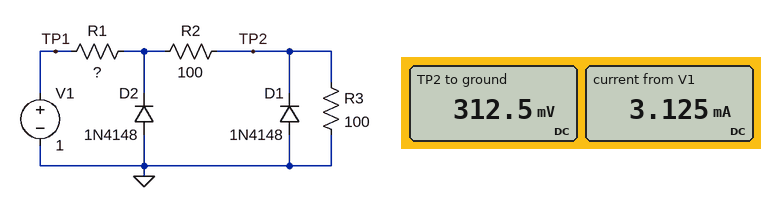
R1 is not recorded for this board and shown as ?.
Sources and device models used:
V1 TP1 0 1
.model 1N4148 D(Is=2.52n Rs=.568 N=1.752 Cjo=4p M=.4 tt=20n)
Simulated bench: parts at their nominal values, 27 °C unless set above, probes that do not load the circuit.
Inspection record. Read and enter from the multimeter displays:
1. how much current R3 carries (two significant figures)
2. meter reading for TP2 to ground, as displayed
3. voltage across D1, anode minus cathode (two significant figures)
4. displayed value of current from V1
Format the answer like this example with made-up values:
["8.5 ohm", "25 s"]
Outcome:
["3.1 mA", "312.5 mV", "-310 mV", "3.125 mA"]
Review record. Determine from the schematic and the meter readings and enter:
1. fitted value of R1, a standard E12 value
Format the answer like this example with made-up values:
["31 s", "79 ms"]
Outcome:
["120 Ω"]
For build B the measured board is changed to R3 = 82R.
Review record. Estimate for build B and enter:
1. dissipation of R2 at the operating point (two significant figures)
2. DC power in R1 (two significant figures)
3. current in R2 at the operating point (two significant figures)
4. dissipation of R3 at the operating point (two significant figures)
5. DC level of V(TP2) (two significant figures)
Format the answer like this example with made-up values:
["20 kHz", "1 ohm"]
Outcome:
["1.1 mW", "1.3 mW", "3.3 mA", "900 µW", "270 mV"]
